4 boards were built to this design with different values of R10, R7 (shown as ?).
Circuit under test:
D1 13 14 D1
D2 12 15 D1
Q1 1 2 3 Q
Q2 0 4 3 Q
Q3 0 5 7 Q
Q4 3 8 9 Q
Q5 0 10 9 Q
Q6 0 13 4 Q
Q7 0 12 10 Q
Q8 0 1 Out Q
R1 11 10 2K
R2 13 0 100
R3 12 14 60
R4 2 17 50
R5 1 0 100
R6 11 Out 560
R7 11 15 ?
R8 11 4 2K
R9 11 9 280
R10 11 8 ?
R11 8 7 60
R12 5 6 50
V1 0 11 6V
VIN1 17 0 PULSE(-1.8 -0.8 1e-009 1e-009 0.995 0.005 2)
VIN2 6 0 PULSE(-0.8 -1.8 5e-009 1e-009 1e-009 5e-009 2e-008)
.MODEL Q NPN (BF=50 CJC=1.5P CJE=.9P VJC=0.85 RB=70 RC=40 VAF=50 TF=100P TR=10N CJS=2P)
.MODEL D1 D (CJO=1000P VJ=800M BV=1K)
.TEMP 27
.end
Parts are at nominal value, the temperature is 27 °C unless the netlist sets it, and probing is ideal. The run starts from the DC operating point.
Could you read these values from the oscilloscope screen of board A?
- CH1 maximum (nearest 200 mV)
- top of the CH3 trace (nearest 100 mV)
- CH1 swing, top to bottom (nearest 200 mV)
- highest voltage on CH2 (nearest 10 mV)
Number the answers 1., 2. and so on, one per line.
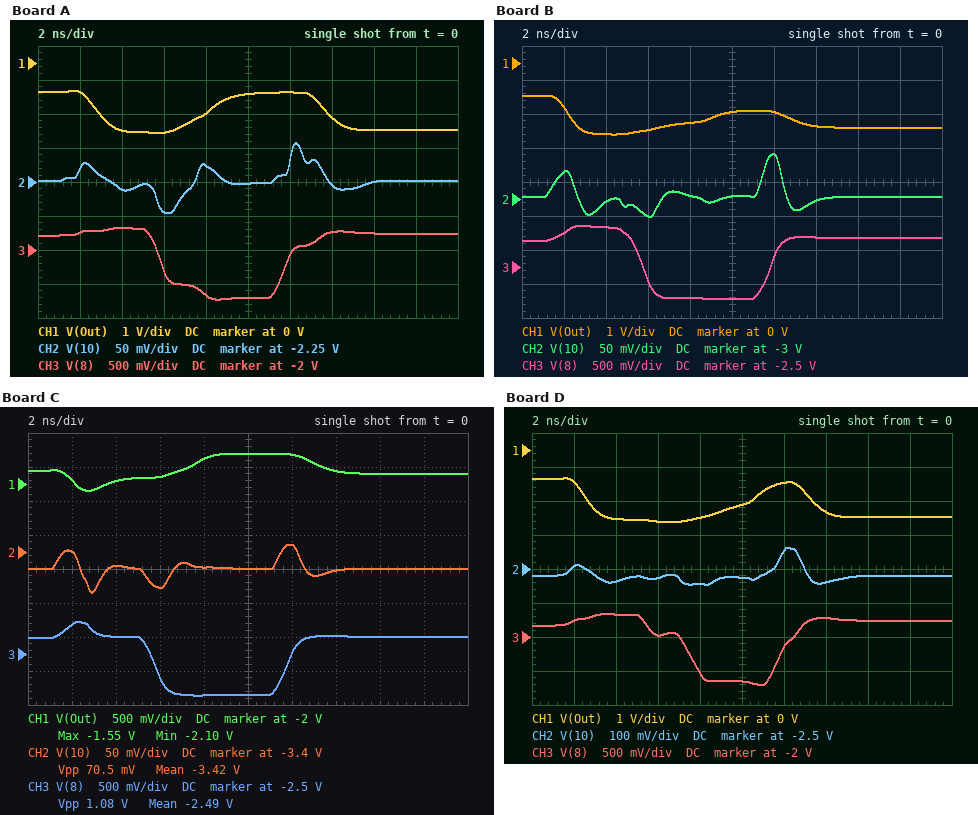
1. -800 mV
2. -1.7 V
3. 1.2 V
4. -2.19 V
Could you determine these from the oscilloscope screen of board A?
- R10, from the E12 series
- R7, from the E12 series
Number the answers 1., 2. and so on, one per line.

1. 1.8 kΩ
2. 820 Ω
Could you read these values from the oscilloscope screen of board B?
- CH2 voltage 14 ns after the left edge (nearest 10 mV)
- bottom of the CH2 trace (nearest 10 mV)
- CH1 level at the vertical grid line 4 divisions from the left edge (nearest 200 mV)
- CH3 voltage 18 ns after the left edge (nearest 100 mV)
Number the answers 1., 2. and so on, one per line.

1. -3.00 V
2. -3.03 V
3. -1.8 V
4. -2.1 V
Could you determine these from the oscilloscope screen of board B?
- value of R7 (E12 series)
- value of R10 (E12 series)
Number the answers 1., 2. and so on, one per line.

1. 330 Ω
2. 560 Ω
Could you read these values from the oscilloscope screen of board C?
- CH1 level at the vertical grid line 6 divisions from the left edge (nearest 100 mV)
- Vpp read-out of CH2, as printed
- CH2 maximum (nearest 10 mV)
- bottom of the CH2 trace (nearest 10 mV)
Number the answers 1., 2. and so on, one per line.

1. -1.6 V
2. 70.5 mV
3. -3.39 V
4. -3.46 V
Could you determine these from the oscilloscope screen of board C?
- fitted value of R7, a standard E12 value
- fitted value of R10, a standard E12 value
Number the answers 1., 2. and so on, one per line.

1. 220 Ω
2. 390 Ω
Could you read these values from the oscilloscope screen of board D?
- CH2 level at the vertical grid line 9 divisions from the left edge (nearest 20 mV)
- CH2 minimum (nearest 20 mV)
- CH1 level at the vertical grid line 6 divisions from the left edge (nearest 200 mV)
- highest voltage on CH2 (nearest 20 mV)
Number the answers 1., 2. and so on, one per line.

1. -2.52 V
2. -2.54 V
3. -1.0 V
4. -2.44 V
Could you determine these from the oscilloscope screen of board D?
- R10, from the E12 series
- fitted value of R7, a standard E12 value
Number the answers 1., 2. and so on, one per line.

1. 1.8 kΩ
2. 560 Ω
